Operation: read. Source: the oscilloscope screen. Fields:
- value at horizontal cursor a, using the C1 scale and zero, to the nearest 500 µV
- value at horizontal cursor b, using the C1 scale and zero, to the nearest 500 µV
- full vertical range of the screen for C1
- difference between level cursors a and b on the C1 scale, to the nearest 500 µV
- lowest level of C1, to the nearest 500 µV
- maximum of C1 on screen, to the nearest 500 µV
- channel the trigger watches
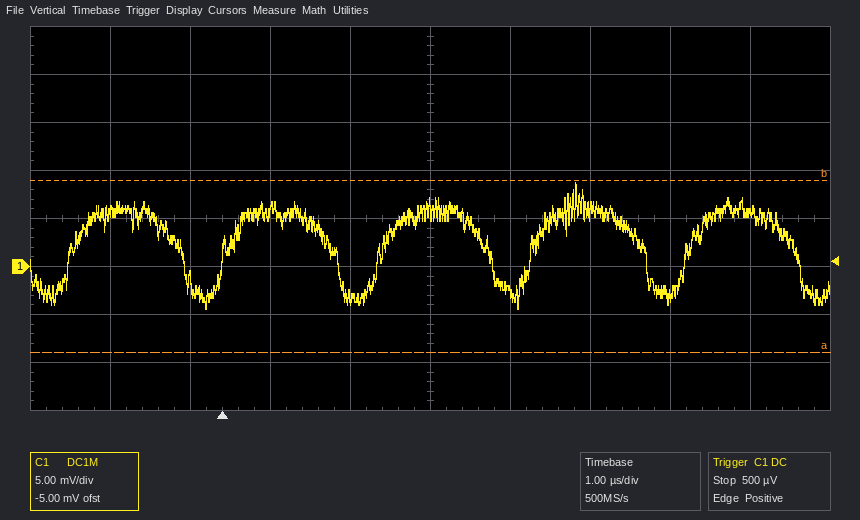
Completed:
-9.0 mV
9.0 mV
40 mV
18.0 mV
-4.5 mV
9.0 mV
C1
